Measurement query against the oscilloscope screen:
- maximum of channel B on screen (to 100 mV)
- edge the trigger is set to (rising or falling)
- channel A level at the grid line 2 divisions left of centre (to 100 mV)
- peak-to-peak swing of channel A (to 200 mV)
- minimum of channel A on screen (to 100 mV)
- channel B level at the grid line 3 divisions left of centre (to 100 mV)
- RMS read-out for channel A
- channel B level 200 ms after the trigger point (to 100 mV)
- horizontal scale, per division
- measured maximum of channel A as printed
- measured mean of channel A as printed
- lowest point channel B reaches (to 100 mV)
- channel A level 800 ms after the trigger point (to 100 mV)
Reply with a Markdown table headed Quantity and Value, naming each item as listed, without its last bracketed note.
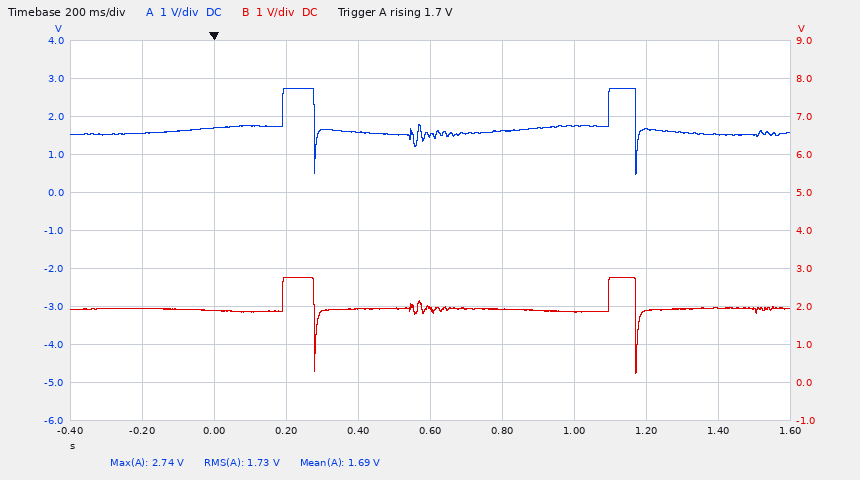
| Quantity | Value |
|---|---|
| maximum of channel B on screen | 2.8 V |
| edge the trigger is set to | rising |
| channel A level at the grid line 2 divisions left of centre | 2.7 V |
| peak-to-peak swing of channel A | 2.2 V |
| minimum of channel A on screen | 500 mV |
| channel B level at the grid line 3 divisions left of centre | 1.9 V |
| RMS read-out for channel A | 1.73 V |
| channel B level 200 ms after the trigger point | 2.7 V |
| horizontal scale, per division | 200 ms |
| measured maximum of channel A as printed | 2.74 V |
| measured mean of channel A as printed | 1.69 V |
| lowest point channel B reaches | 200 mV |
| channel A level 800 ms after the trigger point | 1.6 V |
